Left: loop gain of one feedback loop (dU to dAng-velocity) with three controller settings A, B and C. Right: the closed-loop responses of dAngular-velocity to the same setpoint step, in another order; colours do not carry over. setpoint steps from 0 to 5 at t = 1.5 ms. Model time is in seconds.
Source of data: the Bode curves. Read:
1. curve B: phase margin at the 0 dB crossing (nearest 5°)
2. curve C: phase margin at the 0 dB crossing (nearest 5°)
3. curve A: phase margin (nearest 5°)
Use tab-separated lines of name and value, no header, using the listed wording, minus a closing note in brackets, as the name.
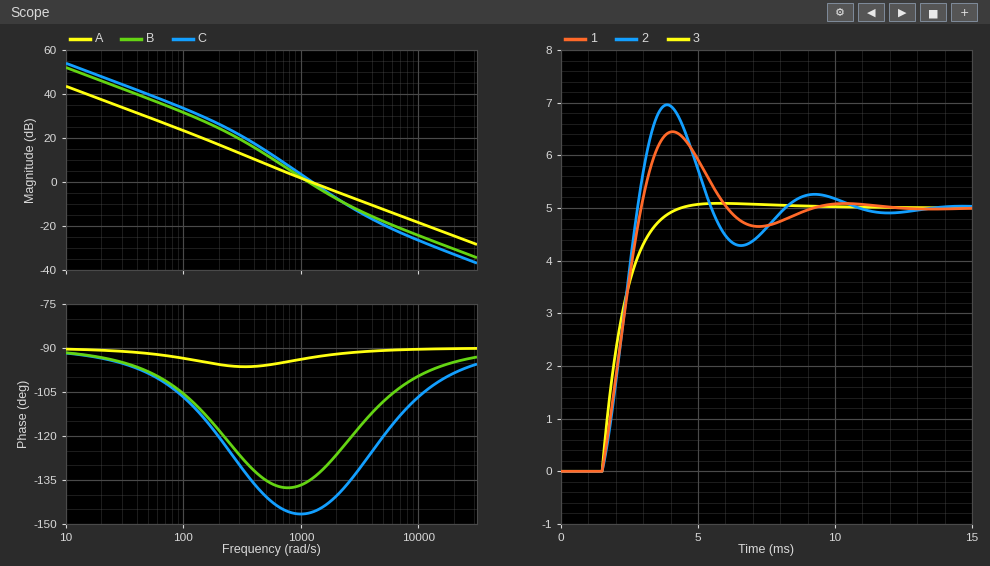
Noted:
curve B: phase margin at the 0 dB crossing	45°
curve C: phase margin at the 0 dB crossing	35°
curve A: phase margin	85°
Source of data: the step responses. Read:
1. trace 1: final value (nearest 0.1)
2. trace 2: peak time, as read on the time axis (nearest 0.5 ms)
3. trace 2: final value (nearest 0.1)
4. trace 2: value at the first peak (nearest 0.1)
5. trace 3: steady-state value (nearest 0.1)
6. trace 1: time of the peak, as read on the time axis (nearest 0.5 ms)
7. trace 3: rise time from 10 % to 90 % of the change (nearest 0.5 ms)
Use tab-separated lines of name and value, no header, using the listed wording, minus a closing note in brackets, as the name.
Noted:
trace 1: final value	5.0
trace 2: peak time, as read on the time axis	4.0 ms
trace 2: final value	5.0
trace 2: value at the first peak	7.0
trace 3: steady-state value	5.0
trace 1: time of the peak, as read on the time axis	4.0 ms
trace 3: rise time from 10 % to 90 % of the change	1.5 ms
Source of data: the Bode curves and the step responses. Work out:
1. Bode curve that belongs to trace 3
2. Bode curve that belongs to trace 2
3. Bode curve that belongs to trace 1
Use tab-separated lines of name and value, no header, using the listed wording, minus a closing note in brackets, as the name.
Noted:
Bode curve that belongs to trace 3	A
Bode curve that belongs to trace 2	C
Bode curve that belongs to trace 1	B
